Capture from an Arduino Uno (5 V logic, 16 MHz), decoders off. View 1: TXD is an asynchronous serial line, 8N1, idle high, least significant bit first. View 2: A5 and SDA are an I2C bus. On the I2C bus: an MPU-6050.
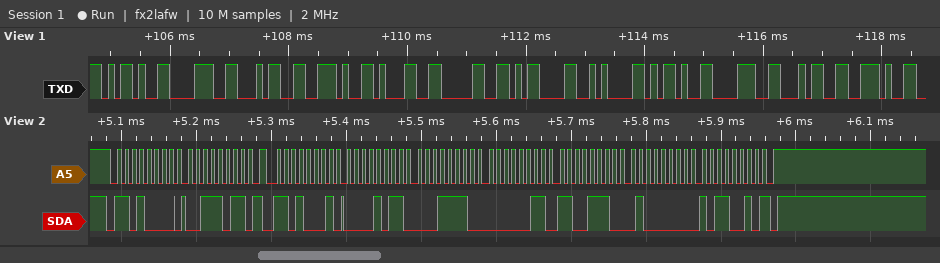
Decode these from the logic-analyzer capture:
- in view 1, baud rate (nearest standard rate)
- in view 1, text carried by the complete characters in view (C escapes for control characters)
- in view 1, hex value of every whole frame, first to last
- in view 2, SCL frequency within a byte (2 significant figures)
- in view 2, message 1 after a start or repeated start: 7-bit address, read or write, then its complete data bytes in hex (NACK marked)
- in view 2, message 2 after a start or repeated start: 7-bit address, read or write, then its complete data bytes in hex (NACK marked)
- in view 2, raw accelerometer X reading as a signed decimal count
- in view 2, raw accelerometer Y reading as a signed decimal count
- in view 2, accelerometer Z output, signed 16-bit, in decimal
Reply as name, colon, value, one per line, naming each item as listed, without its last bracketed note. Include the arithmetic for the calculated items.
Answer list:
in view 1, baud rate: 9600 baud
in view 1, text carried by the complete characters in view: "-84.10\r\n-84."
in view 1, hex value of every whole frame, first to last: 2D 38 34 2E 31 30 0D 0A 2D 38 34 2E
in view 2, SCL frequency within a byte: 100 kHz
in view 2, message 1 after a start or repeated start: 7-bit address, read or write, then its complete data bytes in hex: 0x68 write: 3B
in view 2, message 2 after a start or repeated start: 7-bit address, read or write, then its complete data bytes in hex: 0x68 read: 0B 1E 03 CE 40 B2 NACK
in view 2, raw accelerometer X reading as a signed decimal count: 0x0B1E = 2846
in view 2, raw accelerometer Y reading as a signed decimal count: 0x03CE = 974
in view 2, accelerometer Z output, signed 16-bit, in decimal: 0x40B2 = 16562
